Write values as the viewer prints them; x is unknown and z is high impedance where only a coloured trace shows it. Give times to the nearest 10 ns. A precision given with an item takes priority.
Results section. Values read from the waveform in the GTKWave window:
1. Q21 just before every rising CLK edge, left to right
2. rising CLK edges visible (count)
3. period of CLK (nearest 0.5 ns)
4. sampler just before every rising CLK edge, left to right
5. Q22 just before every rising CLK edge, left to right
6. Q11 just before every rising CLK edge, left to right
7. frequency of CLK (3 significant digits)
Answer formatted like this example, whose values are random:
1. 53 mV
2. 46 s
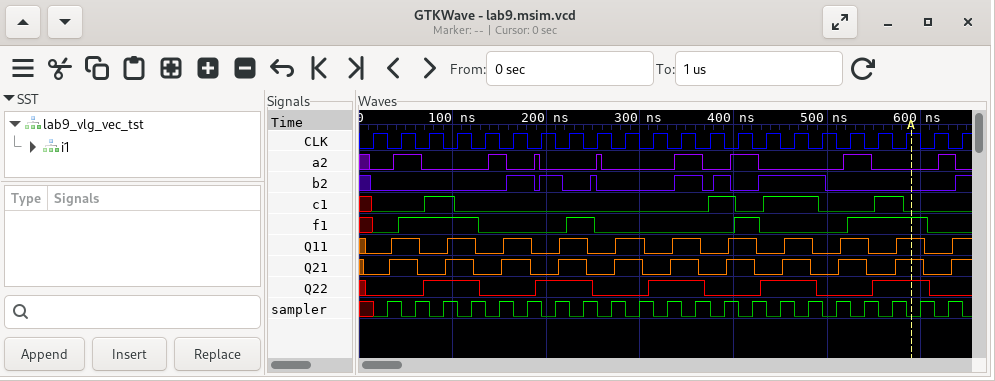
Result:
1. 0 1 0 1 0 1 0 1 0 1 0 1 0 1 0 1 0 1 0 1 0 1
2. 22
3. 30 ns
4. x 1 1 1 1 1 1 1 1 1 1 1 1 1 1 1 1 1 1 1 1 1
5. 0 0 1 1 0 0 1 1 0 0 1 1 0 0 1 1 0 0 1 1 0 0
6. 0 1 0 1 0 1 0 1 0 1 0 1 0 1 0 1 0 1 0 1 0 1
7. 33.3 MHz
